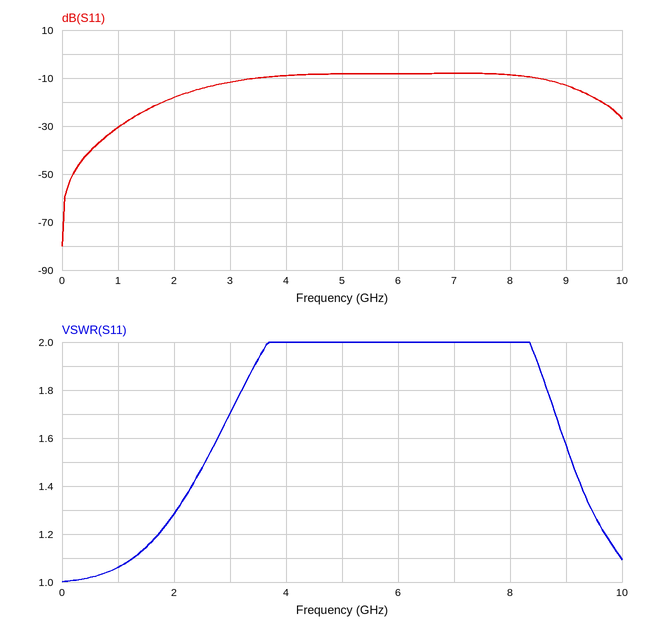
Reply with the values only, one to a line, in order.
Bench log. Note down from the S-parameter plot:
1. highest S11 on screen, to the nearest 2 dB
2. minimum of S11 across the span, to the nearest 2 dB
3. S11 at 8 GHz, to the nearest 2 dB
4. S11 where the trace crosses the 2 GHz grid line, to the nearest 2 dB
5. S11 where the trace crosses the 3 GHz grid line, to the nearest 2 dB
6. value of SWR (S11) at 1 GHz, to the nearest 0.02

-8 dB
-80 dB
-8 dB
-18 dB
-12 dB
1.06
